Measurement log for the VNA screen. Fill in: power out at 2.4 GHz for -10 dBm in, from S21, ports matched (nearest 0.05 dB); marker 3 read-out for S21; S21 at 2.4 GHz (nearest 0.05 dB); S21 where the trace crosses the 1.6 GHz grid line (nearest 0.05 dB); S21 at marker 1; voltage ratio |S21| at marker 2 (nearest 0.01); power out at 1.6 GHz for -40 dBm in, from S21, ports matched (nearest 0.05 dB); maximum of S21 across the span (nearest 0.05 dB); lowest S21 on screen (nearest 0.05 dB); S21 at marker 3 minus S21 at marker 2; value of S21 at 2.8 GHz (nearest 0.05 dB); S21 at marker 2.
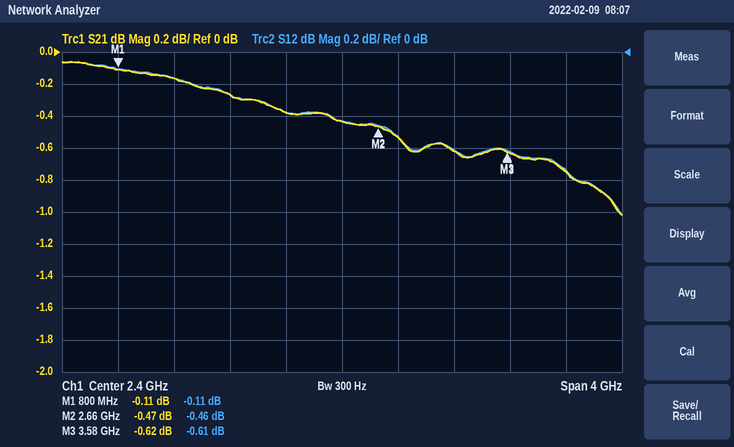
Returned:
-10.45 dBm
-0.62 dB
-0.45 dB
-0.25 dB
-0.11 dB
0.95
-40.25 dBm
-0.05 dB
-1.00 dB
-0.15 dB
-0.55 dB
-0.47 dB
